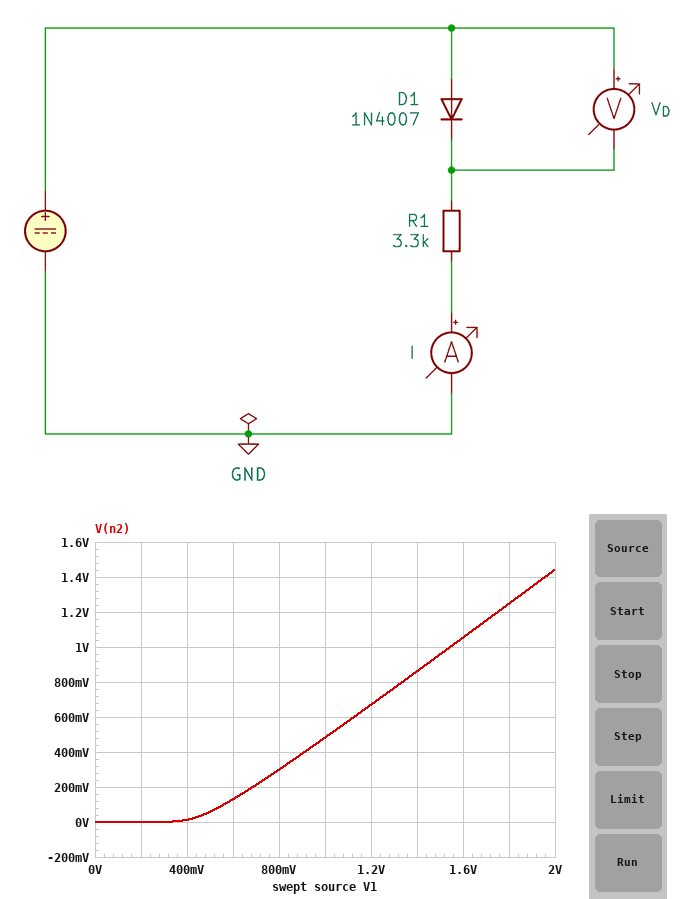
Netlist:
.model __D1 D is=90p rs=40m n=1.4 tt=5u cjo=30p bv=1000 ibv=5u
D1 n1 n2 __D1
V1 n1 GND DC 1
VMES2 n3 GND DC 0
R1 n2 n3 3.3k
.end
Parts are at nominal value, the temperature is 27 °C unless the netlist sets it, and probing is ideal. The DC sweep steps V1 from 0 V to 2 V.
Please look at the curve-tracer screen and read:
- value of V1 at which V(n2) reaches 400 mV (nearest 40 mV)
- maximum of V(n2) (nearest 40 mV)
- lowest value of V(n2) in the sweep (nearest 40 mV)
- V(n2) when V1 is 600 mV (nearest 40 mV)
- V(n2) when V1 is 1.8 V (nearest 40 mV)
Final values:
920 mV
1.44 V
0 V
120 mV
1.24 V
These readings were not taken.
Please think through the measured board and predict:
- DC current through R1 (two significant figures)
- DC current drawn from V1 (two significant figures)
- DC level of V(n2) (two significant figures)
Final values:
150 µA
150 µA
480 mV
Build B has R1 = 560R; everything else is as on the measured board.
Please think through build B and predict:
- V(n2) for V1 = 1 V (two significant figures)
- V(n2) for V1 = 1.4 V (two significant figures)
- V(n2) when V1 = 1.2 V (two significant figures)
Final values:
420 mV
800 mV
610 mV
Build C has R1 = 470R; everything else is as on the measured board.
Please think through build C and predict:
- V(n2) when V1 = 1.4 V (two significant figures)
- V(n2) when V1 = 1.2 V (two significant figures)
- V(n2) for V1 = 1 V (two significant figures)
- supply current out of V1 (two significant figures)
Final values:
790 mV
600 mV
420 mV
890 µA
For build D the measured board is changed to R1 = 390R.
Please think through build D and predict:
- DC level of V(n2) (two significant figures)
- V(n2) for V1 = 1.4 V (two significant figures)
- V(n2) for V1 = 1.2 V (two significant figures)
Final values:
410 mV
790 mV
600 mV
